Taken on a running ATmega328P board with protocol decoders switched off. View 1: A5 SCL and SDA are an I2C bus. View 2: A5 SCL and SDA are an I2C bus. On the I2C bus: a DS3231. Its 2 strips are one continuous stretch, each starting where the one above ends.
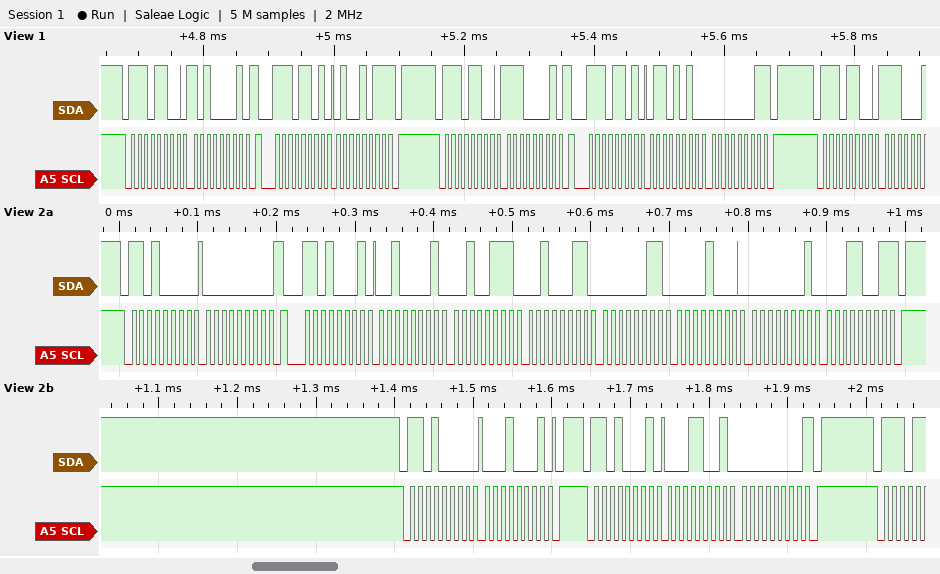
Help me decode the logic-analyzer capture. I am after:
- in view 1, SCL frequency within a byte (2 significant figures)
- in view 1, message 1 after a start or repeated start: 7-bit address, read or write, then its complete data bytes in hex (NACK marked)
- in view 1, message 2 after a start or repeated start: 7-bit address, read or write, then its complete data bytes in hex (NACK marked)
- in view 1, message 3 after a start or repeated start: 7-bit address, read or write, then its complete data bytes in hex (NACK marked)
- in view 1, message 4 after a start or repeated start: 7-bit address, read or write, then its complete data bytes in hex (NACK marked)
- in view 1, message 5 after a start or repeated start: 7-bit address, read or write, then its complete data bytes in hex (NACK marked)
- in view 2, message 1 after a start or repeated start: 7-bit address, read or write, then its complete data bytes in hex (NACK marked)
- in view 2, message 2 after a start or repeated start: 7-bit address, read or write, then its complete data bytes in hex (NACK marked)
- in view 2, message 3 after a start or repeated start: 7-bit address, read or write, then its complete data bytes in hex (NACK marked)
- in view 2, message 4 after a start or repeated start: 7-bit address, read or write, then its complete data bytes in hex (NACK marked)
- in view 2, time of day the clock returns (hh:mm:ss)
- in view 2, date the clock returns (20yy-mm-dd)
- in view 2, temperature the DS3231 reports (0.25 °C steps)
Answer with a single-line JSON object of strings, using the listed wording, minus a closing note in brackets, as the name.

{"in view 1, SCL frequency within a byte": "100 kHz", "in view 1, message 1 after a start or repeated start: 7-bit address, read or write, then its complete data bytes in hex": "0x76 write: A1", "in view 1, message 2 after a start or repeated start: 7-bit address, read or write, then its complete data bytes in hex": "0x76 read: 4B NACK", "in view 1, message 3 after a start or repeated start: 7-bit address, read or write, then its complete data bytes in hex": "0x76 write: E1", "in view 1, message 4 after a start or repeated start: 7-bit address, read or write, then its complete data bytes in hex": "0x76 read: 6A 01 NACK", "in view 1, message 5 after a start or repeated start: 7-bit address, read or write, then its complete data bytes in hex": "0x76 write", "in view 2, message 1 after a start or repeated start: 7-bit address, read or write, then its complete data bytes in hex": "0x68 write: 00", "in view 2, message 2 after a start or repeated start: 7-bit address, read or write, then its complete data bytes in hex": "0x68 read: 21 27 23 03 08 01 19 NACK", "in view 2, message 3 after a start or repeated start: 7-bit address, read or write, then its complete data bytes in hex": "0x68 write: 11", "in view 2, message 4 after a start or repeated start: 7-bit address, read or write, then its complete data bytes in hex": "0x68 read: 19 00 NACK", "in view 2, time of day the clock returns": "23:27:21", "in view 2, date the clock returns": "2019-01-08", "in view 2, temperature the DS3231 reports": "25.00 °C"}
